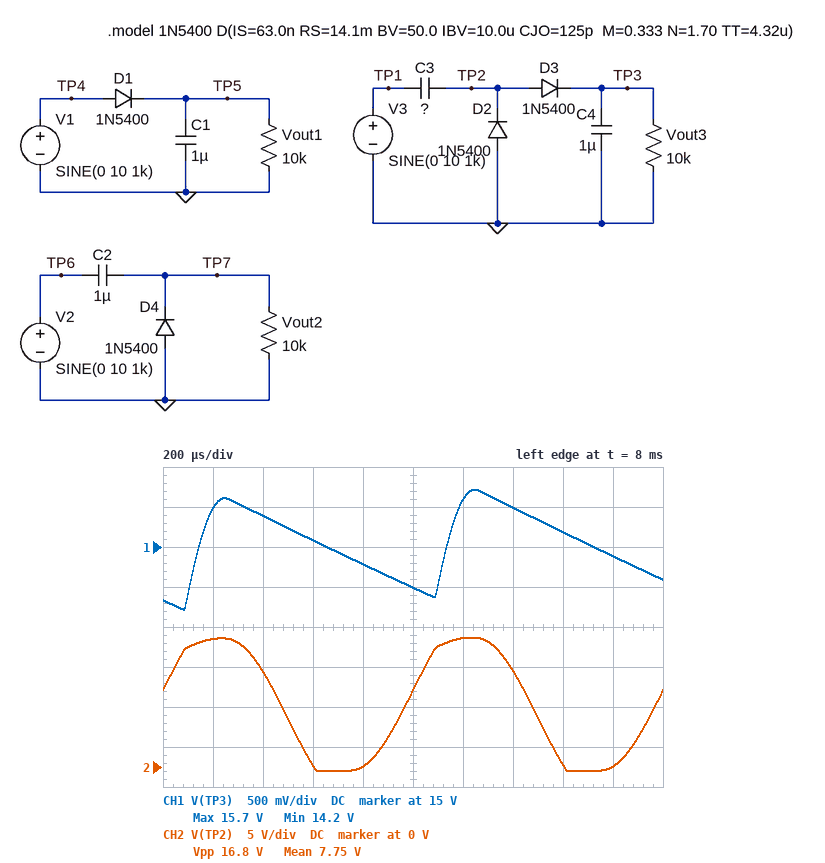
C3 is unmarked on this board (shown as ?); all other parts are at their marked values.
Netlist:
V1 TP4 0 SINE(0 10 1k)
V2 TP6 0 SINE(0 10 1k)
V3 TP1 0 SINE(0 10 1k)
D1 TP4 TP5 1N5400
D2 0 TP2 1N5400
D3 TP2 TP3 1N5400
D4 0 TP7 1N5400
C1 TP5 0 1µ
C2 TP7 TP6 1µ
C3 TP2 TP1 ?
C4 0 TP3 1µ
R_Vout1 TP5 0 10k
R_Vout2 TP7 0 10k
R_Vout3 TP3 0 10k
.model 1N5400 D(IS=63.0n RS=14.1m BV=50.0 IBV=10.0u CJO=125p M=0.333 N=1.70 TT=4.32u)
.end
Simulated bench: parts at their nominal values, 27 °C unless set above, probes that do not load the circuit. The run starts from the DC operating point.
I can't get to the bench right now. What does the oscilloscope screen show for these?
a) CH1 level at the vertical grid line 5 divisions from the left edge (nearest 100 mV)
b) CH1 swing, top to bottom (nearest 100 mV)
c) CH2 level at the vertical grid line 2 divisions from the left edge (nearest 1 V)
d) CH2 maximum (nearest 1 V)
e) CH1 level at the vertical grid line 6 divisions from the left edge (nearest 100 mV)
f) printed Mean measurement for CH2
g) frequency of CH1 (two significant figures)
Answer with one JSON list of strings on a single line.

["14.5 V", "1.5 V", "12 V", "16 V", "15.6 V", "7.75 V", "1.0 kHz"]
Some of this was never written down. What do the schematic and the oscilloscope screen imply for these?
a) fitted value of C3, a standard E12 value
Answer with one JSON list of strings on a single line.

["470 nF"]
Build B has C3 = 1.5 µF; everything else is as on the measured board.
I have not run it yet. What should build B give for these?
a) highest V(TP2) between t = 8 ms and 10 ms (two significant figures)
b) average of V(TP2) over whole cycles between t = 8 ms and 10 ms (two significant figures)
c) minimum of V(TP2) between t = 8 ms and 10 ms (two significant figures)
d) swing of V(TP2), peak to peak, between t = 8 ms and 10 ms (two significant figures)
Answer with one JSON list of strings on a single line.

["18 V", "8.9 V", "-580 mV", "19 V"]
